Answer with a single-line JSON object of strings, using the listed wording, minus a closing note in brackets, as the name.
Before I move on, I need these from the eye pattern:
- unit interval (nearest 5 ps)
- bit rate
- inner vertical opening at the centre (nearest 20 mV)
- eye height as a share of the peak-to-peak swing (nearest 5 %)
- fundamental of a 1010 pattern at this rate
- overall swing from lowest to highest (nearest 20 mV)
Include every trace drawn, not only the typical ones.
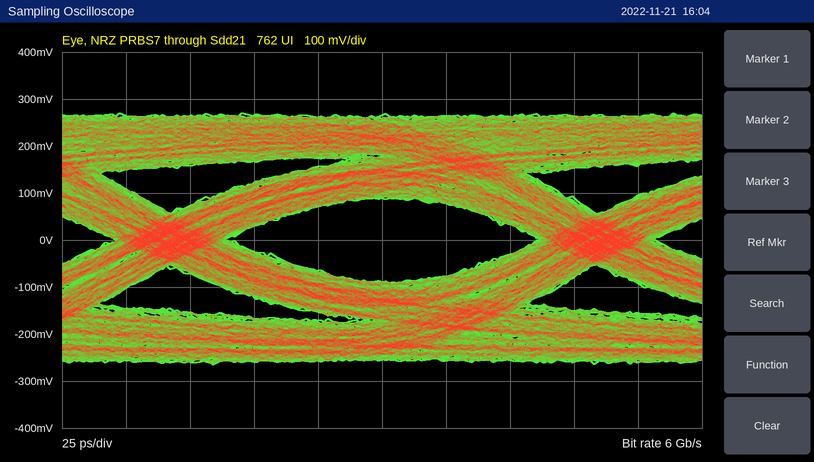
{"unit interval": "165 ps", "bit rate": "6 Gb/s", "inner vertical opening at the centre": "180 mV", "eye height as a share of the peak-to-peak swing": "35 %", "fundamental of a 1010 pattern at this rate": "3 GHz", "overall swing from lowest to highest": "540 mV"}
